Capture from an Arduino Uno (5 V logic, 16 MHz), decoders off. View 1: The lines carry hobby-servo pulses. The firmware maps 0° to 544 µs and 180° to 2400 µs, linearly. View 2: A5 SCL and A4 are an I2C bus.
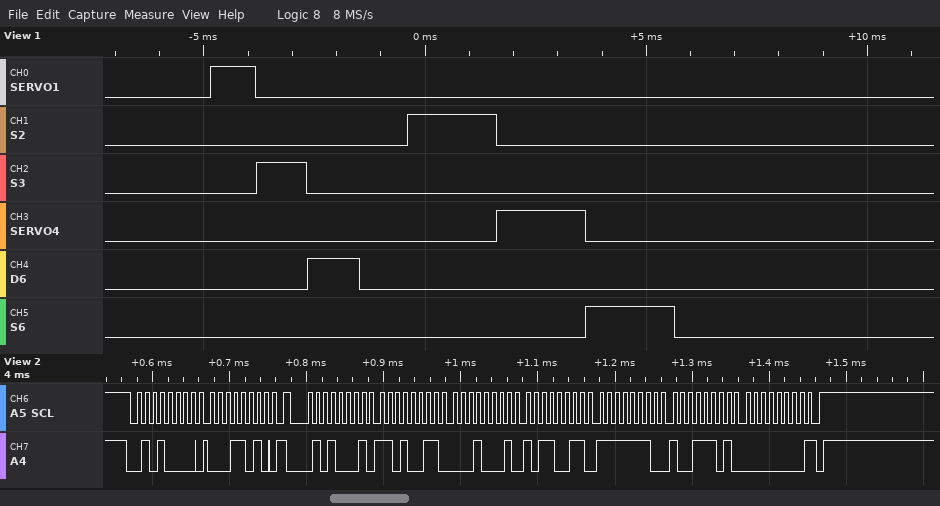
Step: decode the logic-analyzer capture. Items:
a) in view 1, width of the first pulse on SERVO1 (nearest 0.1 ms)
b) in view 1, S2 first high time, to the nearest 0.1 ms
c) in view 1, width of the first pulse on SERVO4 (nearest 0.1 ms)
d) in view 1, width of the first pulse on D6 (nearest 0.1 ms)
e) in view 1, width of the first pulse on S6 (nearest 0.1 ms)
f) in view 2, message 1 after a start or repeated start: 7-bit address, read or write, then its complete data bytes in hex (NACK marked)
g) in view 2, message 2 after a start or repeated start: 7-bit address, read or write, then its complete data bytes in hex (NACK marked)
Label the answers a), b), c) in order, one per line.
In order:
a) 1.0 ms
b) 2.0 ms
c) 2.0 ms
d) 1.2 ms
e) 2.0 ms
f) 0x28 write: 1A
g) 0x28 read: D3 11 B3 FE 9D 00 NACK
